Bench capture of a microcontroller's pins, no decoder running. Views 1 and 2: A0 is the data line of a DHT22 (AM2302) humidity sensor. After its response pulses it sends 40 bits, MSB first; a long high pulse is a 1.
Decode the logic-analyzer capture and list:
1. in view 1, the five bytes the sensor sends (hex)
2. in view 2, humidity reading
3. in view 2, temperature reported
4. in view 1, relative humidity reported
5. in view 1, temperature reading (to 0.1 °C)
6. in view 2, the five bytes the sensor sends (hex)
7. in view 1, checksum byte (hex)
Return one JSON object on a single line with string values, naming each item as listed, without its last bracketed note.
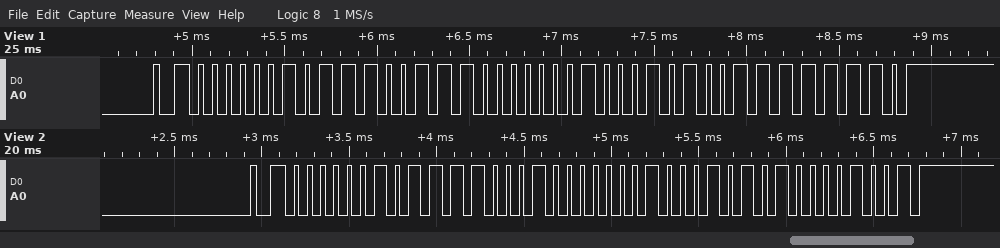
{"in view 1, the five bytes the sensor sends": "02 E7 01 14 FE", "in view 2, humidity reading": "75.3 %", "in view 2, temperature reported": "27.7 °C", "in view 1, relative humidity reported": "74.3 %", "in view 1, temperature reading": "27.6 °C", "in view 2, the five bytes the sensor sends": "02 F1 01 15 09", "in view 1, checksum byte": "0xFE"}
